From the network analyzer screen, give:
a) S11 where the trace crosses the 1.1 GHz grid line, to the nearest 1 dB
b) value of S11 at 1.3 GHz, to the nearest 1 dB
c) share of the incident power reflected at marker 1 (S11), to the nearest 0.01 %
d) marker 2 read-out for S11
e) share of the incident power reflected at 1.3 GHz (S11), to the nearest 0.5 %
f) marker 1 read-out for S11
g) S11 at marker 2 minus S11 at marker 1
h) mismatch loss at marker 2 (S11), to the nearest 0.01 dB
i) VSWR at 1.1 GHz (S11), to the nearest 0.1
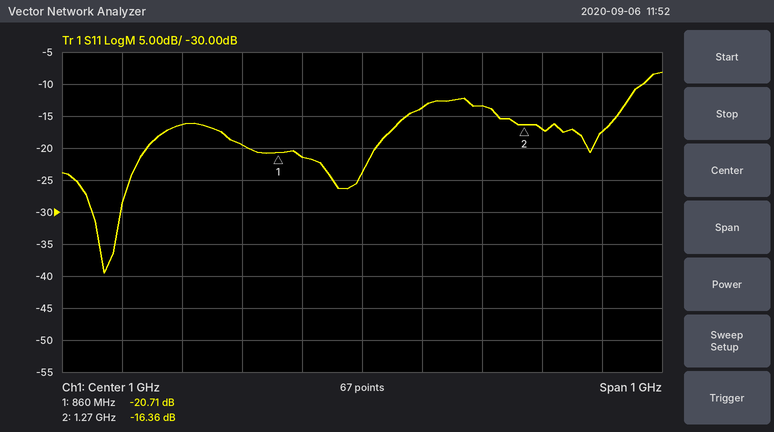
-14 dB
-17 dB
0.85 %
-16.36 dB
2.0 %
-20.71 dB
4.35 dB
0.10 dB
1.5
